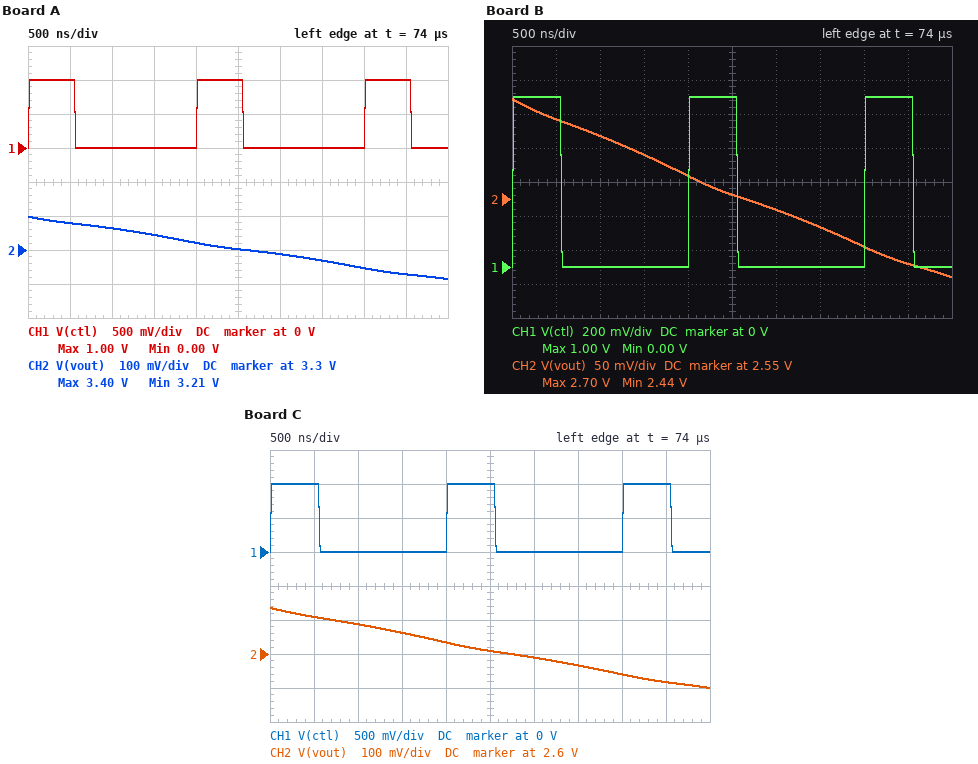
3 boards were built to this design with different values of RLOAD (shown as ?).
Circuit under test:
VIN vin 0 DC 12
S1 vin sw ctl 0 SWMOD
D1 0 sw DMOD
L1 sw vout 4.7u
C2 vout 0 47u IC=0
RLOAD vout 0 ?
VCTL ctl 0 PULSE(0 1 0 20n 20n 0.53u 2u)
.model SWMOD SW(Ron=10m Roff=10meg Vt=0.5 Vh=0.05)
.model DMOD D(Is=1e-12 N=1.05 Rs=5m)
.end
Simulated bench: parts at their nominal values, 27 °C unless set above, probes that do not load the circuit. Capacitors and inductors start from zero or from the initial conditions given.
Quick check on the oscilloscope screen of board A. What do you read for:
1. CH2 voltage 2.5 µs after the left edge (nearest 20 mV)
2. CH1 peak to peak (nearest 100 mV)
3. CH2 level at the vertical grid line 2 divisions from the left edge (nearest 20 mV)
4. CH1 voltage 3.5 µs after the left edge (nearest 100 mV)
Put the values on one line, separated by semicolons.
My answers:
3.30 V; 1.0 V; 3.36 V; 0 V
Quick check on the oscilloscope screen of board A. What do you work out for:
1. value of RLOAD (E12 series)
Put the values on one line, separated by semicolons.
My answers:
1.5 Ω
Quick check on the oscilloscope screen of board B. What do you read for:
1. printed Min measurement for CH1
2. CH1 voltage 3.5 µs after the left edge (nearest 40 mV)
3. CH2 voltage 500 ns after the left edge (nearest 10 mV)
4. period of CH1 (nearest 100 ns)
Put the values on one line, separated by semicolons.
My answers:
0.00 V; 0 V; 2.67 V; 2.0 µs
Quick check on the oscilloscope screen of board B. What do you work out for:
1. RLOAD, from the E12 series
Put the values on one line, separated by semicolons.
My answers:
0.82 Ω
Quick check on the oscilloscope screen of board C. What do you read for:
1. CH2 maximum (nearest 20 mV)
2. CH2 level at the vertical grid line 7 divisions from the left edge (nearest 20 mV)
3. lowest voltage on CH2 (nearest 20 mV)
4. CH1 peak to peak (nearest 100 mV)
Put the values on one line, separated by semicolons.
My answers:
2.74 V; 2.56 V; 2.50 V; 1.0 V
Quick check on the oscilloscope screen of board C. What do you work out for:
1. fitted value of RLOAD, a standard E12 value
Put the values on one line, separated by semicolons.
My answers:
0.68 Ω
